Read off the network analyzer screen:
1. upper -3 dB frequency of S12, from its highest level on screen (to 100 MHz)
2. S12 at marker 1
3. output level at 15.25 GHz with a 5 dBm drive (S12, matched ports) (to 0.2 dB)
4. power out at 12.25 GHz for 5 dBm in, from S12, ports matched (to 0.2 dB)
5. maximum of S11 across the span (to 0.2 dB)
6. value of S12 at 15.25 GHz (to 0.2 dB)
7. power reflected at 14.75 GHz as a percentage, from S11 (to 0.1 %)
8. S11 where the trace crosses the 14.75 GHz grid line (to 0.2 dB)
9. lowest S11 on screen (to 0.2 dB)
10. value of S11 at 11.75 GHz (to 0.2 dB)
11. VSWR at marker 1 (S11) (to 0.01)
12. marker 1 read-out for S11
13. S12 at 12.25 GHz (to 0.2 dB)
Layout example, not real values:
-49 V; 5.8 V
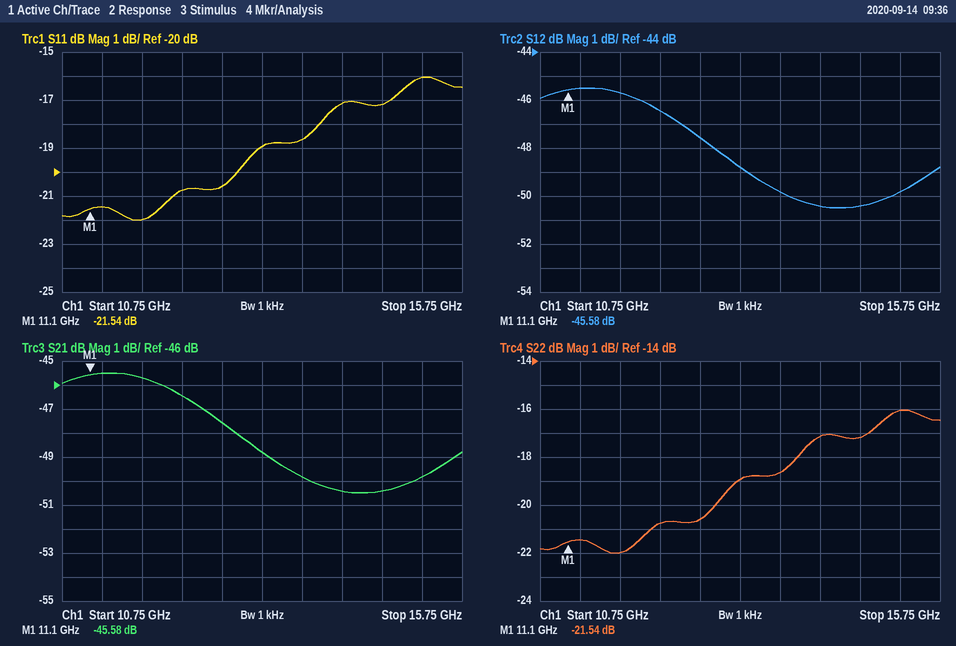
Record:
13.1 GHz; -45.58 dB; -44.8 dBm; -41.4 dBm; -16.0 dB; -49.8 dB; 1.9 %; -17.2 dB; -22.0 dB; -22.0 dB; 1.18; -21.54 dB; -46.4 dB
